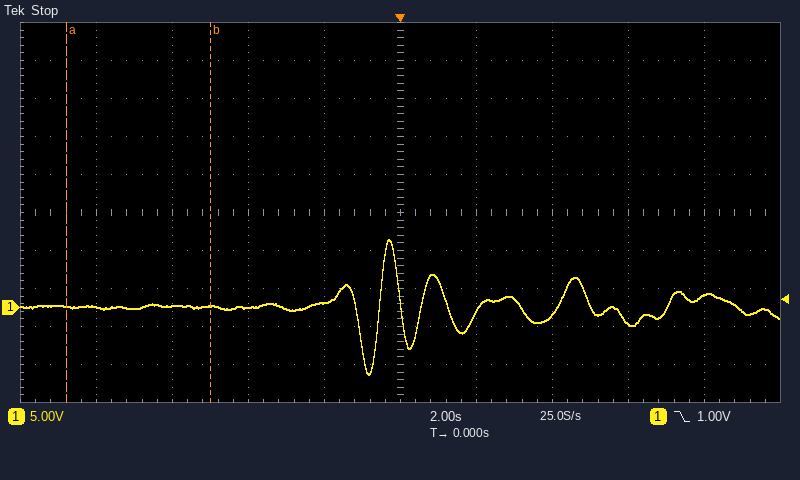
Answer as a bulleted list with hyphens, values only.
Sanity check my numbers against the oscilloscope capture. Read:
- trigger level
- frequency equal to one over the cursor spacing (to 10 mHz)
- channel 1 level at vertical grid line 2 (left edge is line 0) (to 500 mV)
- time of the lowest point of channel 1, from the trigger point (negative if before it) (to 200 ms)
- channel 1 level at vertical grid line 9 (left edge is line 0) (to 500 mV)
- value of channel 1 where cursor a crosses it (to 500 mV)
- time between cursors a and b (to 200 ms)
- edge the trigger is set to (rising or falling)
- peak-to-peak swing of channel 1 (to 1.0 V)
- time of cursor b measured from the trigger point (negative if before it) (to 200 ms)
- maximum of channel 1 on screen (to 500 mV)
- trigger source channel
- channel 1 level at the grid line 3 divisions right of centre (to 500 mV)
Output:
- 1.00 V
- 260 mHz
- 0.0 V
- -800 ms
- 1.5 V
- 0.0 V
- 3.8 s
- falling
- 18.0 V
- -5.0 s
- 9.0 V
- channel 1
- -2.0 V
